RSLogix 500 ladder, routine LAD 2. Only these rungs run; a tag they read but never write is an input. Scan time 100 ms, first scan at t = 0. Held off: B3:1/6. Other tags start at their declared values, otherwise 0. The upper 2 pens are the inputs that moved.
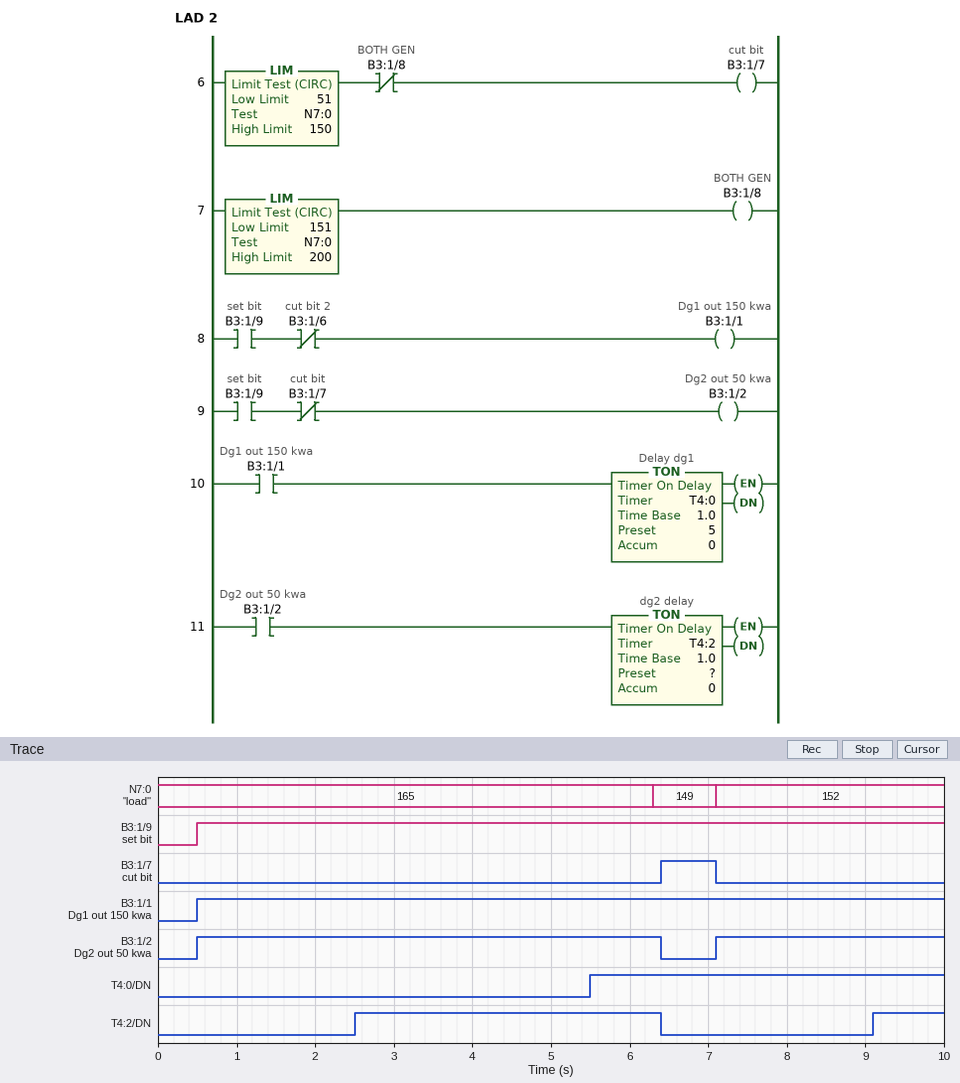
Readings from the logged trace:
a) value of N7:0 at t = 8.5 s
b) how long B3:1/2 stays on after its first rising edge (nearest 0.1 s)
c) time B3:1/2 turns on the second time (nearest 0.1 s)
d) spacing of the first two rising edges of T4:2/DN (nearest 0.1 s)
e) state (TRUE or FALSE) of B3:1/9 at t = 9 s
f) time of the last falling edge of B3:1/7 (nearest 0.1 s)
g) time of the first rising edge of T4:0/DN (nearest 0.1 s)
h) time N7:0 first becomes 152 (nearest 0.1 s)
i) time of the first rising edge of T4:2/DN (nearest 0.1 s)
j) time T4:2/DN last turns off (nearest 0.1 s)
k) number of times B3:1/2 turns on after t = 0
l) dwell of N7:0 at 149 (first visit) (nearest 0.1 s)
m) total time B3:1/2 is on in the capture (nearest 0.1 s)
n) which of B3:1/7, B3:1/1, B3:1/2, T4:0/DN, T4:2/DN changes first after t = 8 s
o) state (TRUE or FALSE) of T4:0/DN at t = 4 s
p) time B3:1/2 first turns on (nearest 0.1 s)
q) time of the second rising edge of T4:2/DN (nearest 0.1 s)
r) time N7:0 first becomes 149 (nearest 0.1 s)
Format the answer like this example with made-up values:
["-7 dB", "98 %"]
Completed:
["152", "5.9 s", "7.1 s", "6.6 s", "TRUE", "7.1 s", "5.5 s", "7.1 s", "2.5 s", "6.4 s", "2", "0.8 s", "8.8 s", "T4:2/DN", "FALSE", "0.5 s", "9.1 s", "6.3 s"]
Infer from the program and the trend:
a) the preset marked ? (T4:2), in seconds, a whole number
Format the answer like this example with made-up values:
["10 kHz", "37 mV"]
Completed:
["2 s"]
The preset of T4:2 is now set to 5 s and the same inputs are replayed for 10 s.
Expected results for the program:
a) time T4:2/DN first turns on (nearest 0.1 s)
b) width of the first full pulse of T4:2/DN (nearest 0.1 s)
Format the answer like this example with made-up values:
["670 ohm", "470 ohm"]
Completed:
["5.5 s", "0.9 s"]
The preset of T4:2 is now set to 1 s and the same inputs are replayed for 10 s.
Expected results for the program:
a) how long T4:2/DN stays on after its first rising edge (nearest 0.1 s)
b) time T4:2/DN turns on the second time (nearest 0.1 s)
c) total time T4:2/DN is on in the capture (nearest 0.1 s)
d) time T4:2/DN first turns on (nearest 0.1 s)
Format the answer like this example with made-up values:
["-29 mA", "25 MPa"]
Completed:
["4.9 s", "8.1 s", "6.8 s", "1.5 s"]
